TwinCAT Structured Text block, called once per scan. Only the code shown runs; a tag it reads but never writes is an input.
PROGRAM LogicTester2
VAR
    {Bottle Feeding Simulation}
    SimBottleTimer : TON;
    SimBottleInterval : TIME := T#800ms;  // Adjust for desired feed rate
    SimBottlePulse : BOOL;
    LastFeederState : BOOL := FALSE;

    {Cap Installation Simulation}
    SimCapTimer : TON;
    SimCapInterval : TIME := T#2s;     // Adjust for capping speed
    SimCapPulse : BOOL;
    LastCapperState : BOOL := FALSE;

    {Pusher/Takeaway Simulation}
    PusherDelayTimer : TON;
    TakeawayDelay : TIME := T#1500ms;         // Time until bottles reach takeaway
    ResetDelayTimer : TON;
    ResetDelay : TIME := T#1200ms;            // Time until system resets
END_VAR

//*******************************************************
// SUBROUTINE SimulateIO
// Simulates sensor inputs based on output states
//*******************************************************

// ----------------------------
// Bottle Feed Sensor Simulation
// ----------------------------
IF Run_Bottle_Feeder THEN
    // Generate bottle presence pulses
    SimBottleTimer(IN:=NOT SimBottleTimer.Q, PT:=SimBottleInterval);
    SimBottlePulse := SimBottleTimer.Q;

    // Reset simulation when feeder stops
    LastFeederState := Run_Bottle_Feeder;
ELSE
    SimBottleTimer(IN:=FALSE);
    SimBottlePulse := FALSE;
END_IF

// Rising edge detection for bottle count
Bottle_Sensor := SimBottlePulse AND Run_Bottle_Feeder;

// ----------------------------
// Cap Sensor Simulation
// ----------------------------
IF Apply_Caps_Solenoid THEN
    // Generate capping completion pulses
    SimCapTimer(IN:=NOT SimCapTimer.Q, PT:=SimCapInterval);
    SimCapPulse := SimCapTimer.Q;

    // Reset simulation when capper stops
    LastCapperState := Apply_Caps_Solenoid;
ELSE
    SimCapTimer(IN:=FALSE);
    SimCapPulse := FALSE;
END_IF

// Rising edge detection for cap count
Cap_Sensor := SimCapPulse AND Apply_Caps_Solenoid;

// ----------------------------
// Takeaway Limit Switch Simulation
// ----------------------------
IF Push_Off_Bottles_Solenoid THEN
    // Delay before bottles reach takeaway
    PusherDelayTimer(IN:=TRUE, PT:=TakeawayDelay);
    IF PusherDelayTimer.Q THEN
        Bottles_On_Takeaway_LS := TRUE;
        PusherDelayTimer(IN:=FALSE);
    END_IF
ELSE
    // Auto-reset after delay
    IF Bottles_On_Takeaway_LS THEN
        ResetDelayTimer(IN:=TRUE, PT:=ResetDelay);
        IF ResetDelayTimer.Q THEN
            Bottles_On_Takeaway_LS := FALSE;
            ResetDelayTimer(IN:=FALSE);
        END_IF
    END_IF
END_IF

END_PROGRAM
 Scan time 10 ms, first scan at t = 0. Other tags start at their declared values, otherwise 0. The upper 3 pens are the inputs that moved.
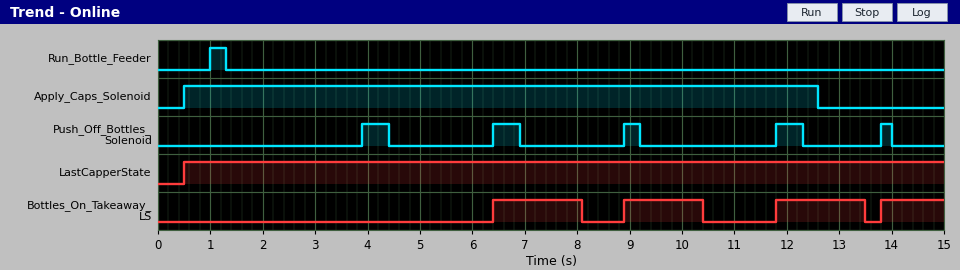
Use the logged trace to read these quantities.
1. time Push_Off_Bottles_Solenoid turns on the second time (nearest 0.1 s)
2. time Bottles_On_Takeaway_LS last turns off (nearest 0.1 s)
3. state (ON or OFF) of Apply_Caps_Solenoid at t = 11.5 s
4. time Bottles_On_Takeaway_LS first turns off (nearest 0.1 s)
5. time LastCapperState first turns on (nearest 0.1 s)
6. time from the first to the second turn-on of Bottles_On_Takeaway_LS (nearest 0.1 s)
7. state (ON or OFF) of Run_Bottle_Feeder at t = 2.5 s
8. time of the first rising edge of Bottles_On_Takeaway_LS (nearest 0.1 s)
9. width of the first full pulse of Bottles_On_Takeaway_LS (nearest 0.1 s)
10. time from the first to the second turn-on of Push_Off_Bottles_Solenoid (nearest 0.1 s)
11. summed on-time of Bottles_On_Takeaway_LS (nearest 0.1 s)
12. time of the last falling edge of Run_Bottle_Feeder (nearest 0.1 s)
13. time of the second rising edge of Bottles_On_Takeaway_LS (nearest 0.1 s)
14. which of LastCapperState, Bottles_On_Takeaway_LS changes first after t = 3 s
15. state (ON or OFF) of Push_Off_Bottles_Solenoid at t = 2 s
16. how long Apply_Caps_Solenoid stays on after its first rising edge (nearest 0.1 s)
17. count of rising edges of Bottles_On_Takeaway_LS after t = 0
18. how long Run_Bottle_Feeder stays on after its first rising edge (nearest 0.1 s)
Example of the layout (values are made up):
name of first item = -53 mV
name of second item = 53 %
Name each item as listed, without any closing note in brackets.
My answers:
time Push_Off_Bottles_Solenoid turns on the second time = 6.4 s
time Bottles_On_Takeaway_LS last turns off = 13.5 s
state (ON or OFF) of Apply_Caps_Solenoid at t = 11.5 s = ON
time Bottles_On_Takeaway_LS first turns off = 8.1 s
time LastCapperState first turns on = 0.5 s
time from the first to the second turn-on of Bottles_On_Takeaway_LS = 2.5 s
state (ON or OFF) of Run_Bottle_Feeder at t = 2.5 s = OFF
time of the first rising edge of Bottles_On_Takeaway_LS = 6.4 s
width of the first full pulse of Bottles_On_Takeaway_LS = 1.7 s
time from the first to the second turn-on of Push_Off_Bottles_Solenoid = 2.5 s
summed on-time of Bottles_On_Takeaway_LS = 6.1 s
time of the last falling edge of Run_Bottle_Feeder = 1.3 s
time of the second rising edge of Bottles_On_Takeaway_LS = 8.9 s
which of LastCapperState, Bottles_On_Takeaway_LS changes first after t = 3 s = Bottles_On_Takeaway_LS
state (ON or OFF) of Push_Off_Bottles_Solenoid at t = 2 s = OFF
how long Apply_Caps_Solenoid stays on after its first rising edge = 12.1 s
count of rising edges of Bottles_On_Takeaway_LS after t = 0 = 4
how long Run_Bottle_Feeder stays on after its first rising edge = 0.3 s
